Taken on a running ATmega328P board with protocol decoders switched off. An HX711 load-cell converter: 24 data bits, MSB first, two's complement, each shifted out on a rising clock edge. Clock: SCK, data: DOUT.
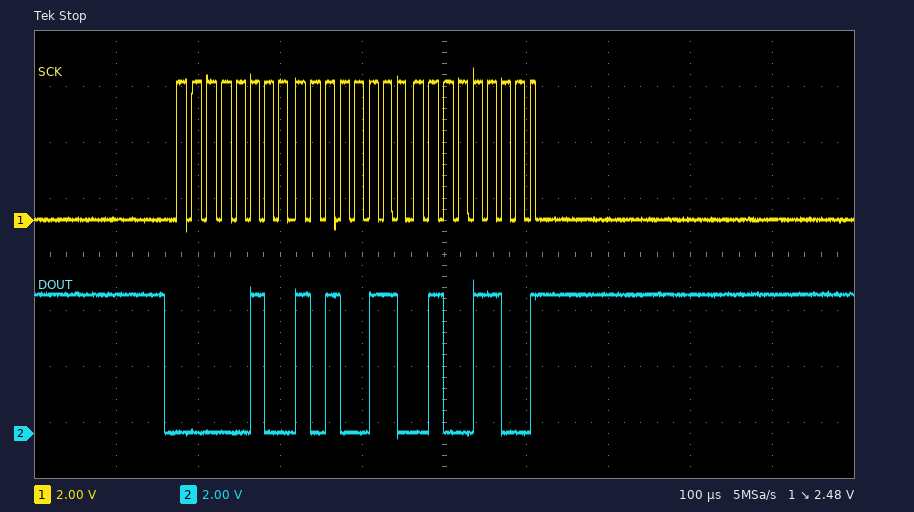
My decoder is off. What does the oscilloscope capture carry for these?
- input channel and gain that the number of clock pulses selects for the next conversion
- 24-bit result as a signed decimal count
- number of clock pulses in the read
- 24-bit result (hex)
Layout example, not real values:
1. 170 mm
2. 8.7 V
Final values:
1. channel A, gain 128
2. 304716
3. 25
4. 0x04A64C
